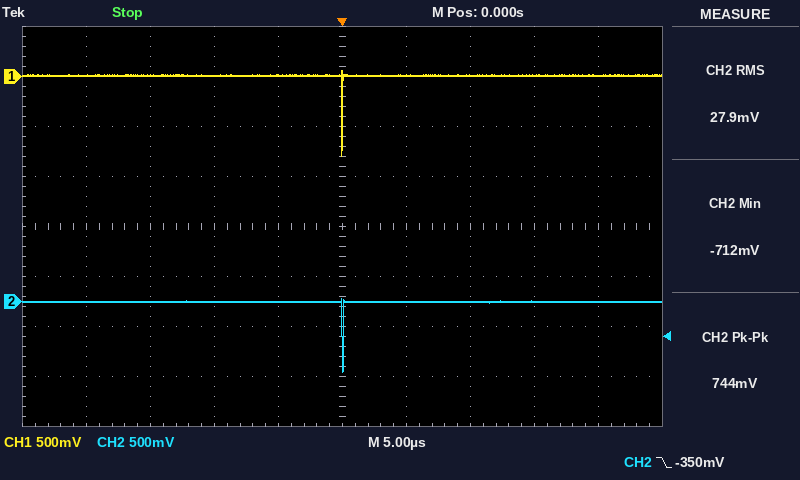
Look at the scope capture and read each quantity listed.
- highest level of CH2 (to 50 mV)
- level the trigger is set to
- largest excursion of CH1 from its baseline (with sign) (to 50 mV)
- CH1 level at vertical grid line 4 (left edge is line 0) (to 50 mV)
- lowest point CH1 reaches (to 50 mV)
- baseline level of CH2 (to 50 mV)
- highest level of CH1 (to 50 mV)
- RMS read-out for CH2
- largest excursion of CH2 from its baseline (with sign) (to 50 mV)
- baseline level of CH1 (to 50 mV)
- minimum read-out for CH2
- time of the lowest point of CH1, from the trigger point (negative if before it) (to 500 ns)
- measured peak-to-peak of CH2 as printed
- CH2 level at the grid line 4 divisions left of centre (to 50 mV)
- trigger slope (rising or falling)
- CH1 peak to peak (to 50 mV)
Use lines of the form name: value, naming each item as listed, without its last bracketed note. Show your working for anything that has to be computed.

highest level of CH2: 50 mV
level the trigger is set to: -350 mV
largest excursion of CH1 from its baseline (with sign): -800 mV − (0 mV) = -800 mV
CH1 level at vertical grid line 4 (left edge is line 0): 0 mV
lowest point CH1 reaches: -800 mV
baseline level of CH2: 0 mV
highest level of CH1: 50 mV
RMS read-out for CH2: 27.9 mV
largest excursion of CH2 from its baseline (with sign): -700 mV
baseline level of CH1: 0 mV
minimum read-out for CH2: -712 mV
time of the lowest point of CH1, from the trigger point (negative if before it): 0.0 µs
measured peak-to-peak of CH2 as printed: 744 mV
CH2 level at the grid line 4 divisions left of centre: 0 mV
trigger slope: falling
CH1 peak to peak: 50 mV − (-800 mV) = 850 mV
